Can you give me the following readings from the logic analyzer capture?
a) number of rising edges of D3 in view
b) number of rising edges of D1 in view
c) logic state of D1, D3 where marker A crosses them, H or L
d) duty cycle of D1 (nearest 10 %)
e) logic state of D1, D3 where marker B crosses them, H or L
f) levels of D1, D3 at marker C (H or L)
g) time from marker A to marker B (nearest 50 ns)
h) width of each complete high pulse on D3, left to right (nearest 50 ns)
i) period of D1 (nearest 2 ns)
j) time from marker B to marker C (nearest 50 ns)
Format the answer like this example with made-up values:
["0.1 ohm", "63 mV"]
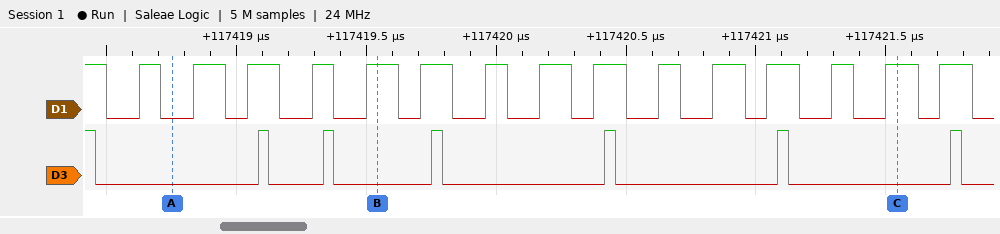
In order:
["6", "15", "D1=L, D3=L", "50 %", "D1=H, D3=L", "D1=H, D3=L", "800 ns", "50 ns, 50 ns, 50 ns, 50 ns, 50 ns, 50 ns", "220 ns", "2000 ns"]
